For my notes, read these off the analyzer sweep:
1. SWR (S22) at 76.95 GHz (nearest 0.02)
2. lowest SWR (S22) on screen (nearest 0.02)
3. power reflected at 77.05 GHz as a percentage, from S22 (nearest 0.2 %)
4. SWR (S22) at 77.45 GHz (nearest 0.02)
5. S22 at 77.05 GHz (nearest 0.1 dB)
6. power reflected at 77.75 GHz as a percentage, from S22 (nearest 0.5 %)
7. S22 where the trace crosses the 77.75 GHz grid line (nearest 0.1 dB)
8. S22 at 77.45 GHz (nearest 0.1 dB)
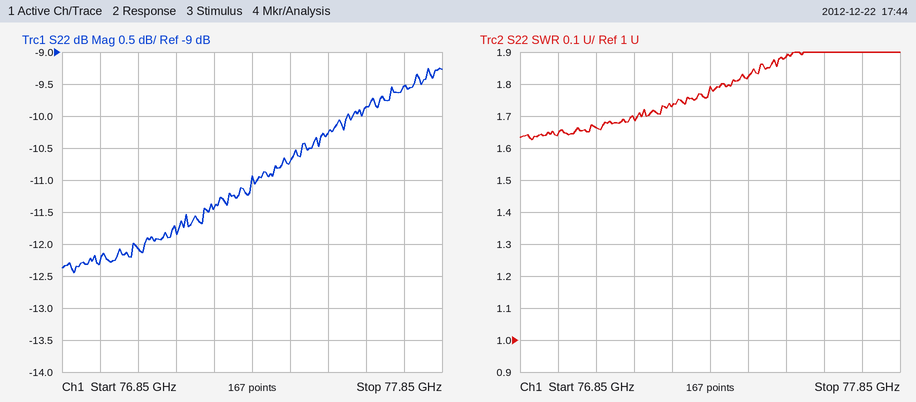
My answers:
1.64
1.62
6.2 %
1.82
-12.1 dB
11.0 %
-9.5 dB
-10.7 dB
